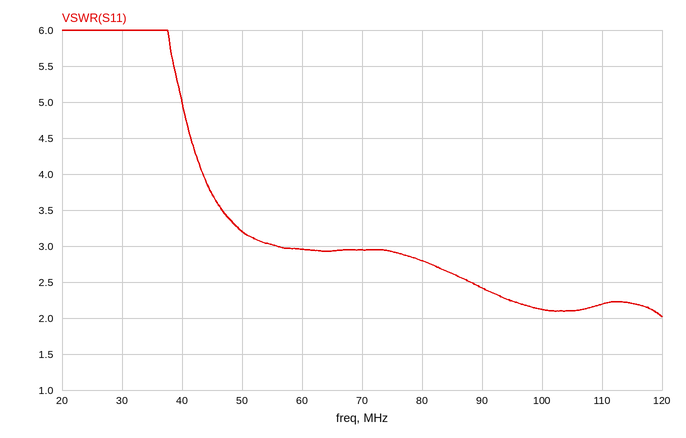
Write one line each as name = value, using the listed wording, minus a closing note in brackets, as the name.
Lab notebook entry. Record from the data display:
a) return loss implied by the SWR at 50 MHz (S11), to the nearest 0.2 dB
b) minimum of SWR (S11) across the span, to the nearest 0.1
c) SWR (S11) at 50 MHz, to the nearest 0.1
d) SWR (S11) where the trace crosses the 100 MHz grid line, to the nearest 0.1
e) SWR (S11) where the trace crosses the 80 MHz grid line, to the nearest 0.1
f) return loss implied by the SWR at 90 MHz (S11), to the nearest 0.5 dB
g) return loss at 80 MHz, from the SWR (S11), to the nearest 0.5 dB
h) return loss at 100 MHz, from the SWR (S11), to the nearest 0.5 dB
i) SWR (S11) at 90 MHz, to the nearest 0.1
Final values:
return loss implied by the SWR at 50 MHz (S11), to the nearest 0.2 dB = 5.6 dB
minimum of SWR (S11) across the span, to the nearest 0.1 = 2.0
SWR (S11) at 50 MHz, to the nearest 0.1 = 3.2
SWR (S11) where the trace crosses the 100 MHz grid line, to the nearest 0.1 = 2.1
SWR (S11) where the trace crosses the 80 MHz grid line, to the nearest 0.1 = 2.8
return loss implied by the SWR at 90 MHz (S11), to the nearest 0.5 dB = 7.5 dB
return loss at 80 MHz, from the SWR (S11), to the nearest 0.5 dB = 6.5 dB
return loss at 100 MHz, from the SWR (S11), to the nearest 0.5 dB = 9.0 dB
SWR (S11) at 90 MHz, to the nearest 0.1 = 2.4
